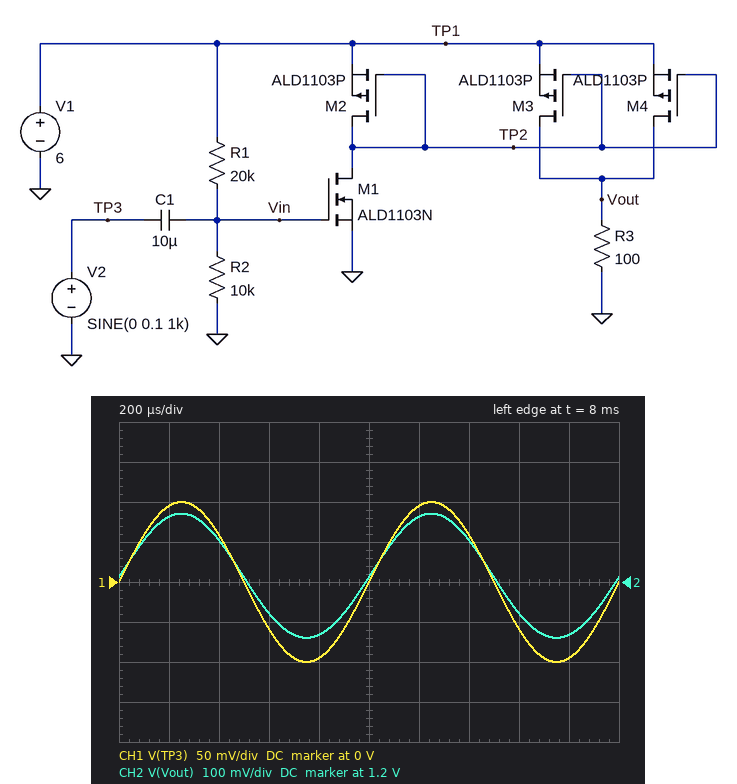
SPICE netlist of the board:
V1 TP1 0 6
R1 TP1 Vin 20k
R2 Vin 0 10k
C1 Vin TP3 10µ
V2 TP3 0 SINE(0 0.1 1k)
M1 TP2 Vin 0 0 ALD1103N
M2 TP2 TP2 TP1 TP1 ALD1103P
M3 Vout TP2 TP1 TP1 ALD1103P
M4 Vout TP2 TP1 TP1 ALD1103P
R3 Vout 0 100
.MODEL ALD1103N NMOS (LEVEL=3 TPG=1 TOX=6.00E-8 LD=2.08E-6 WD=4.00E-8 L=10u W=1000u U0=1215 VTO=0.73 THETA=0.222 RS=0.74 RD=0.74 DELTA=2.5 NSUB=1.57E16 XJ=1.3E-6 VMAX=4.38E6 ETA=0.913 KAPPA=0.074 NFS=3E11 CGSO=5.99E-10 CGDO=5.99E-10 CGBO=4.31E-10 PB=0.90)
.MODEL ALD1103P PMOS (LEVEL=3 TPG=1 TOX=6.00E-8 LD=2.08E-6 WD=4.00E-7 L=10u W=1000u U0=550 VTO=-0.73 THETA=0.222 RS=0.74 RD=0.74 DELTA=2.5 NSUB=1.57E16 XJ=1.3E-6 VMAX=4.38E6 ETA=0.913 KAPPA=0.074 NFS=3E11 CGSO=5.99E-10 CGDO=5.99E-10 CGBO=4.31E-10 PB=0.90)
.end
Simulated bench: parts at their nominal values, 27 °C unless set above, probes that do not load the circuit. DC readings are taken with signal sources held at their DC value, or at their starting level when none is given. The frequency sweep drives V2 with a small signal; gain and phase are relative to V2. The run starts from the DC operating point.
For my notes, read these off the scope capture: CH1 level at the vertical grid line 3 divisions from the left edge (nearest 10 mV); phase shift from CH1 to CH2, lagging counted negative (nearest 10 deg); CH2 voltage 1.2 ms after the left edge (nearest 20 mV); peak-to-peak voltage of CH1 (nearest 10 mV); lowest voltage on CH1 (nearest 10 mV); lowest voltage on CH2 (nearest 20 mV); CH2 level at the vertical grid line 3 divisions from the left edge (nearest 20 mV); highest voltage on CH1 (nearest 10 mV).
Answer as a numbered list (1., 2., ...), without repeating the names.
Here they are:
1. -60 mV
2. 0 deg
3. 1.36 V
4. 200 mV
5. -100 mV
6. 1.06 V
7. 1.12 V
8. 100 mV
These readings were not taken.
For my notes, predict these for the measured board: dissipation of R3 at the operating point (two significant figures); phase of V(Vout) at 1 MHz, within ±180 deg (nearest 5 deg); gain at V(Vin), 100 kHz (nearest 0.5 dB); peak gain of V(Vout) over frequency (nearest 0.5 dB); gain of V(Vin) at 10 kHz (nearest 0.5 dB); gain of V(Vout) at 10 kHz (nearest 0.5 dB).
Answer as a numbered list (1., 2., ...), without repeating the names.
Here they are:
1. 15 mW
2. 0 deg
3. 0 dB
4. 4.0 dB
5. 0 dB
6. 4.0 dB
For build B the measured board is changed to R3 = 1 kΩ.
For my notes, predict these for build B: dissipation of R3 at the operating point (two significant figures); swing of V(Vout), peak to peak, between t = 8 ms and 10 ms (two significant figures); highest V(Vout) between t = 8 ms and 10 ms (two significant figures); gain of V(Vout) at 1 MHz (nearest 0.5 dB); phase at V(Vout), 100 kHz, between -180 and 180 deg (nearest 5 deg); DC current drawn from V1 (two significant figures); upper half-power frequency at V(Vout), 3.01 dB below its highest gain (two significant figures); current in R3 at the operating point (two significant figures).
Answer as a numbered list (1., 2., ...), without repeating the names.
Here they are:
1. 31 mW
2. 60 mV
3. 5.6 V
4. -10.5 dB
5. 0 deg
6. 12 mA
7. 140 MHz
8. 5.6 mA
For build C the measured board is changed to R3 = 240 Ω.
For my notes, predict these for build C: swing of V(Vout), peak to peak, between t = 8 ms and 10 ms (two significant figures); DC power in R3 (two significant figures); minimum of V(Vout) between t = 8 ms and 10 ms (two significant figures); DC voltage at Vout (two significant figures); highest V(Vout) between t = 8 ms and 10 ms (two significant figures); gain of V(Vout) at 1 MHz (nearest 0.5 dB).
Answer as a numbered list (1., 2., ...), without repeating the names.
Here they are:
1. 740 mV
2. 35 mW
3. 2.5 V
4. 2.9 V
5. 3.3 V
6. 11.5 dB
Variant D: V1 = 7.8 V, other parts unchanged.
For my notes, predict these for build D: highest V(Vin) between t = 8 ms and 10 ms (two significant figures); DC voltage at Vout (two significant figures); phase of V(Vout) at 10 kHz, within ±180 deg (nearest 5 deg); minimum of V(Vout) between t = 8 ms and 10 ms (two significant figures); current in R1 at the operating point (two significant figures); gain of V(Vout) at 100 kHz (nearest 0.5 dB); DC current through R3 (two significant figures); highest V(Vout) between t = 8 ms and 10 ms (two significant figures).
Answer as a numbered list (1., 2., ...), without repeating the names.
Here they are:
1. 2.7 V
2. 2.3 V
3. 0 deg
4. 2.1 V
5. 260 µA
6. 6.0 dB
7. 23 mA
8. 2.5 V
